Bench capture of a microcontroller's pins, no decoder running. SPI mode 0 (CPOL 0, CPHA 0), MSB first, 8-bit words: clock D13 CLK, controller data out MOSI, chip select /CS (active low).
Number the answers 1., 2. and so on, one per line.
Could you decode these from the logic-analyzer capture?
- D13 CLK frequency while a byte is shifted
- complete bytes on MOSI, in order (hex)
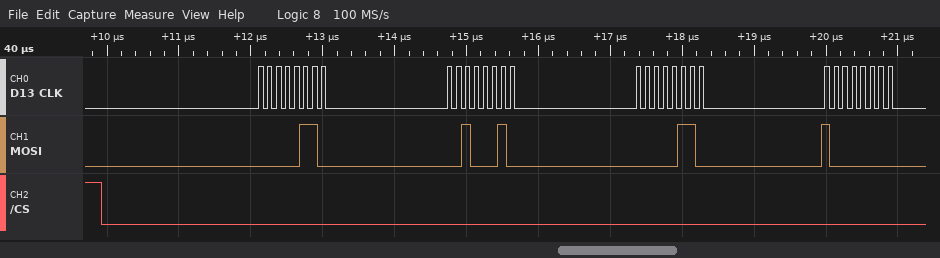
1. 8 MHz
2. 06 22 06 80
